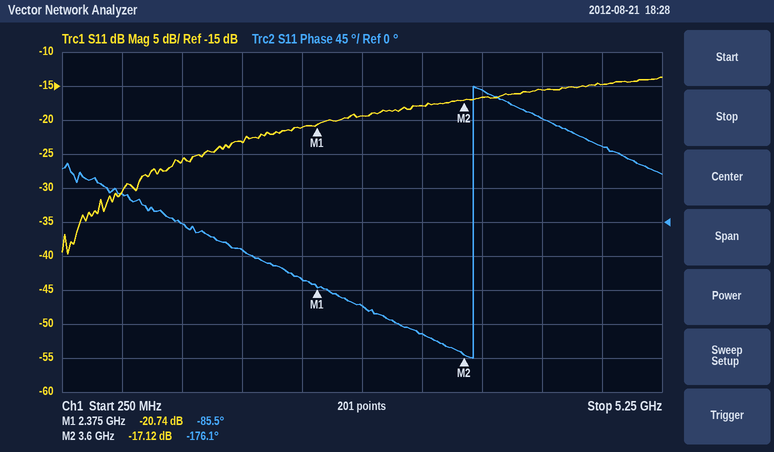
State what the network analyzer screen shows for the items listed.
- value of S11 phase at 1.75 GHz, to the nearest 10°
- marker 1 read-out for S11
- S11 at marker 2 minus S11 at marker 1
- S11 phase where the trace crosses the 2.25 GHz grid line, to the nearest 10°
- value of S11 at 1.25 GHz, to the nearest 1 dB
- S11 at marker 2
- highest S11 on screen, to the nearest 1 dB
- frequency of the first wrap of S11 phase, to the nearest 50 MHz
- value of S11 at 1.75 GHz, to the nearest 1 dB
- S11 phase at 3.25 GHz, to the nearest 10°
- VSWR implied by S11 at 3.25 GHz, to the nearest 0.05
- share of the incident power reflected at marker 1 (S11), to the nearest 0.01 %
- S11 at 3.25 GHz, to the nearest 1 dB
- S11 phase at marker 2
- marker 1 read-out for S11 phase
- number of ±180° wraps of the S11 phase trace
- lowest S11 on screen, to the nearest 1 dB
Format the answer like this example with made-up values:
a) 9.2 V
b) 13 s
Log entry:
a) -40°
b) -20.74 dB
c) 3.62 dB
d) -80°
e) -26 dB
f) -17.12 dB
g) -14 dB
h) 3.70 GHz
i) -23 dB
j) -150°
k) 1.30
l) 0.84 %
m) -18 dB
n) -176.1°
o) -85.5°
p) 1
q) -40 dB
